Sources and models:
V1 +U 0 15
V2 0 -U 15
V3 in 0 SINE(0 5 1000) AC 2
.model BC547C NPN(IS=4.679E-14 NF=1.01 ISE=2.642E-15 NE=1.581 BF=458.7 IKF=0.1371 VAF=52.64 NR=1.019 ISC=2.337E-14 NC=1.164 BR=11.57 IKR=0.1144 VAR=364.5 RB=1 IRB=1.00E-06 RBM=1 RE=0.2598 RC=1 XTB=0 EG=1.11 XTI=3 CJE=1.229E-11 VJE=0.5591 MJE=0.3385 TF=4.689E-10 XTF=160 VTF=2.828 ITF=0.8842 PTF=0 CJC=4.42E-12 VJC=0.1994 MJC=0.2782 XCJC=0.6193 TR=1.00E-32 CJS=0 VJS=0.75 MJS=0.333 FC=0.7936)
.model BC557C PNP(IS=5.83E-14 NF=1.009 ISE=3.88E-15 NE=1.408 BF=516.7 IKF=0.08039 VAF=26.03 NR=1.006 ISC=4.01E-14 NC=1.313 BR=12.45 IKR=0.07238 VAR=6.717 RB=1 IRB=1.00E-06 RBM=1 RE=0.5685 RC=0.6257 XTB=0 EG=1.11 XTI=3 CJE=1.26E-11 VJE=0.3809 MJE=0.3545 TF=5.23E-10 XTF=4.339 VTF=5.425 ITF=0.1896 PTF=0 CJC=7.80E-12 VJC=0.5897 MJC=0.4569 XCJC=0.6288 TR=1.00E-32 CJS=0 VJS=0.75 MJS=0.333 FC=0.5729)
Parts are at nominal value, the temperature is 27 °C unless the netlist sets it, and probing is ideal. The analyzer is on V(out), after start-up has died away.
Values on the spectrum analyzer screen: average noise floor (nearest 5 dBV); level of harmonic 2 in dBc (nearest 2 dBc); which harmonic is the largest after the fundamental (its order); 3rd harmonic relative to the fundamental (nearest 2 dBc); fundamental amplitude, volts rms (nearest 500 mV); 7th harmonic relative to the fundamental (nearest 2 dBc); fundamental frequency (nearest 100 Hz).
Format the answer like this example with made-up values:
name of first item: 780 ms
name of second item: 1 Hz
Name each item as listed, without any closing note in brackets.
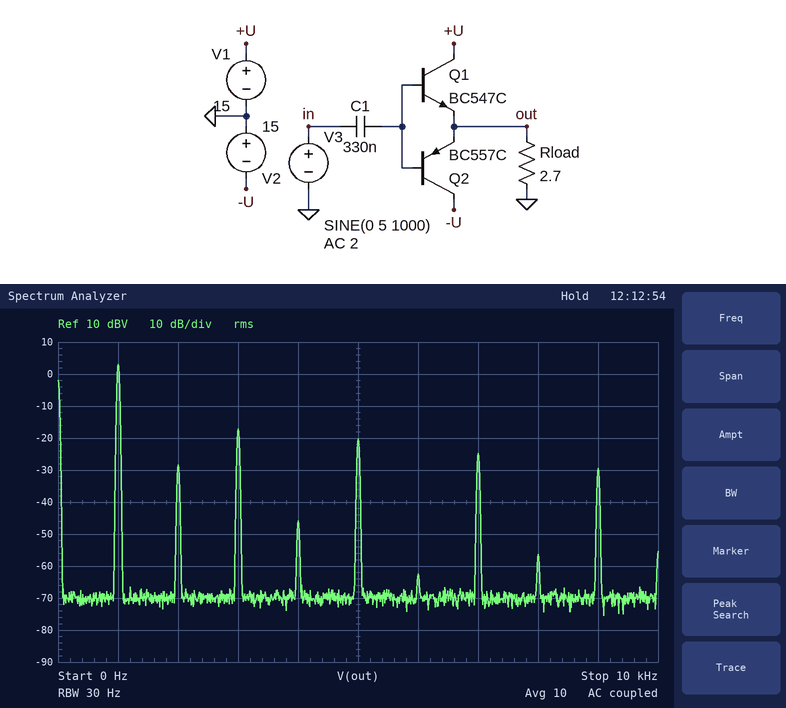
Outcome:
average noise floor: -70 dBV
level of harmonic 2 in dBc: -32 dBc
which harmonic is the largest after the fundamental: 3
3rd harmonic relative to the fundamental: -20 dBc
fundamental amplitude, volts rms: 1.5 V
7th harmonic relative to the fundamental: -28 dBc
fundamental frequency: 1.0 kHz
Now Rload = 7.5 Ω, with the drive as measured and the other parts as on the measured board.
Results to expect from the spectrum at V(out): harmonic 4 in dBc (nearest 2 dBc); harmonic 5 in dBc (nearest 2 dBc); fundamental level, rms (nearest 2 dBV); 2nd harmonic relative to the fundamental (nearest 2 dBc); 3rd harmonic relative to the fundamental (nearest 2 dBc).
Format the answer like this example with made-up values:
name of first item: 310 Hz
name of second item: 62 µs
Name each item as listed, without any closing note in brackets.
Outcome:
harmonic 4 in dBc: -48 dBc
harmonic 5 in dBc: -28 dBc
fundamental level, rms: 8 dBV
2nd harmonic relative to the fundamental: -36 dBc
3rd harmonic relative to the fundamental: -22 dBc
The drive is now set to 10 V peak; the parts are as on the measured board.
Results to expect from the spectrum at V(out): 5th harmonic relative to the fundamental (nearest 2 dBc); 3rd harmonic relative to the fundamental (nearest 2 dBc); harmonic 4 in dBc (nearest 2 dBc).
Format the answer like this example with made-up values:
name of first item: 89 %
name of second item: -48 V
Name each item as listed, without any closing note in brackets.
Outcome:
5th harmonic relative to the fundamental: -26 dBc
3rd harmonic relative to the fundamental: -22 dBc
harmonic 4 in dBc: -44 dBc
